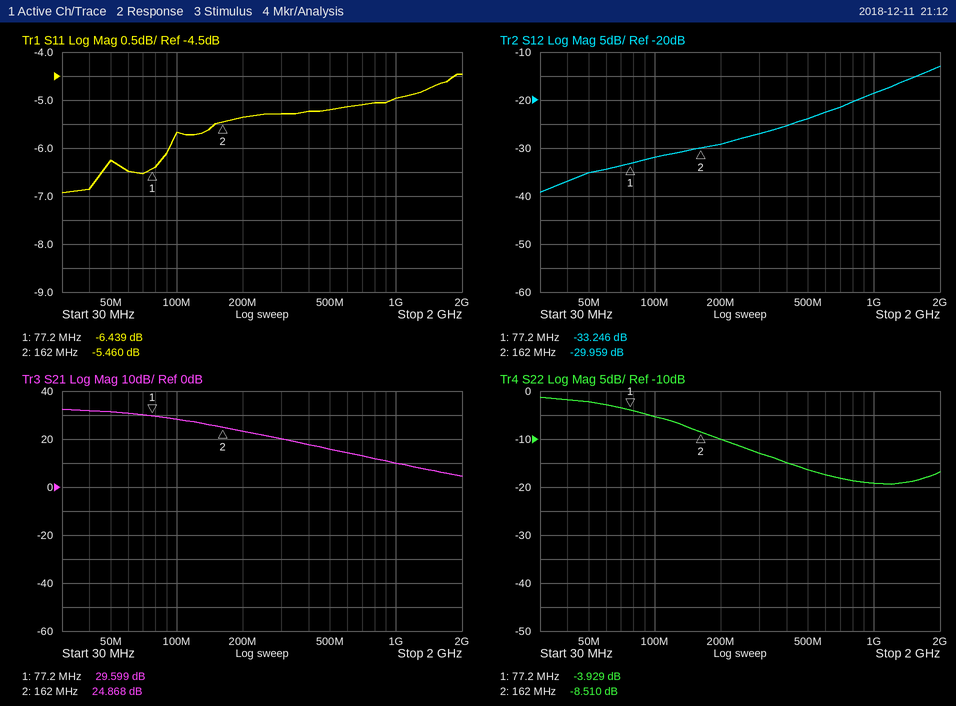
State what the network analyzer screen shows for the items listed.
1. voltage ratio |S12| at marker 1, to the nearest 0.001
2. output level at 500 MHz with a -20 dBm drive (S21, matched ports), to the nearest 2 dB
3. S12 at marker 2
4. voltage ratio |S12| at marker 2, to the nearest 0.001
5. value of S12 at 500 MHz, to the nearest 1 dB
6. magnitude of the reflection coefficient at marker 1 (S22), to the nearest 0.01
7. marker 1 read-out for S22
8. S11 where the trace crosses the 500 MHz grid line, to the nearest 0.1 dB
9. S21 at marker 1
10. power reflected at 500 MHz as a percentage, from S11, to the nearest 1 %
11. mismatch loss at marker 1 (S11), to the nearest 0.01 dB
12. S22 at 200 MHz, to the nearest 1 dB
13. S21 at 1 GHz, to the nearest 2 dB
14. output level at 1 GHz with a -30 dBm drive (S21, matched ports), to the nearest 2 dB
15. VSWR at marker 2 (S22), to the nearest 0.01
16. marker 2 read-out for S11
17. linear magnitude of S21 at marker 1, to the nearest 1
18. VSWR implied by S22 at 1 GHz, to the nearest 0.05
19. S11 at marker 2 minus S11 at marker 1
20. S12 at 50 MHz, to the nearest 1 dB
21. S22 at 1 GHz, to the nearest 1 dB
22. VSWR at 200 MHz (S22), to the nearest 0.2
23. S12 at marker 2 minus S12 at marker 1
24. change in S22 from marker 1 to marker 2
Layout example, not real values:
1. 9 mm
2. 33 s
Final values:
1. 0.022
2. -4 dBm
3. -29.959 dB
4. 0.032
5. -24 dB
6. 0.64
7. -3.929 dB
8. -5.2 dB
9. 29.599 dB
10. 30 %
11. 1.12 dB
12. -10 dB
13. 10 dB
14. -20 dBm
15. 2.20
16. -5.460 dB
17. 30
18. 1.25
19. 0.979 dB
20. -35 dB
21. -19 dB
22. 2.0
23. 3.287 dB
24. -4.581 dB
